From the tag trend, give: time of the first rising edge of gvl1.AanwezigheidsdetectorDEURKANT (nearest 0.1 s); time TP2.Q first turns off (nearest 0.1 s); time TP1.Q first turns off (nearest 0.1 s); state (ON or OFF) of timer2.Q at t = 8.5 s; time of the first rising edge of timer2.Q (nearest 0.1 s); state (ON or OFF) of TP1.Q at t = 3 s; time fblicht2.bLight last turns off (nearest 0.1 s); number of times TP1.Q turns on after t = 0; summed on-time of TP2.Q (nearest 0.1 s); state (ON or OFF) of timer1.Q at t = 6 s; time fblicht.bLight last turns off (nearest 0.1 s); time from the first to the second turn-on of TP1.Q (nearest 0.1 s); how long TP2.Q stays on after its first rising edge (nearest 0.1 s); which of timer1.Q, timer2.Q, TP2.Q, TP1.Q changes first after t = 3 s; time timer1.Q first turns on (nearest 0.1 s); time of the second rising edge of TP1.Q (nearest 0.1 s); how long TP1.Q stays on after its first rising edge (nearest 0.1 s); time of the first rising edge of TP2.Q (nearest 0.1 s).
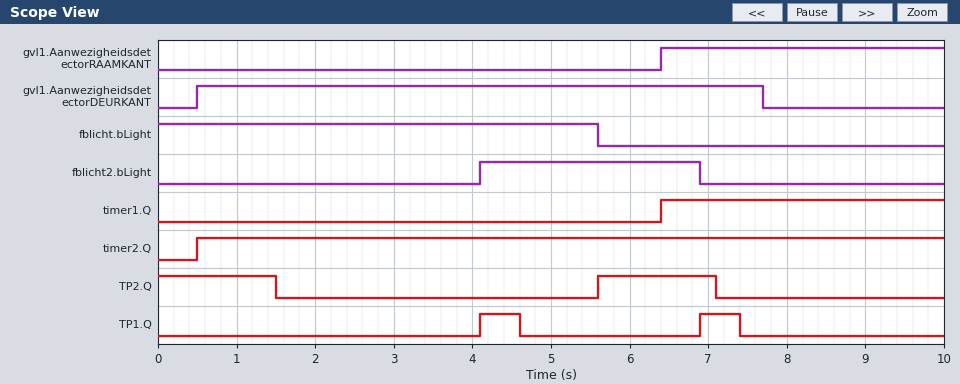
0.5 s
1.5 s
4.6 s
ON
0.5 s
OFF
6.9 s
2
3.0 s
OFF
5.6 s
2.8 s
1.5 s
TP1.Q
6.4 s
6.9 s
0.5 s
5.6 s
